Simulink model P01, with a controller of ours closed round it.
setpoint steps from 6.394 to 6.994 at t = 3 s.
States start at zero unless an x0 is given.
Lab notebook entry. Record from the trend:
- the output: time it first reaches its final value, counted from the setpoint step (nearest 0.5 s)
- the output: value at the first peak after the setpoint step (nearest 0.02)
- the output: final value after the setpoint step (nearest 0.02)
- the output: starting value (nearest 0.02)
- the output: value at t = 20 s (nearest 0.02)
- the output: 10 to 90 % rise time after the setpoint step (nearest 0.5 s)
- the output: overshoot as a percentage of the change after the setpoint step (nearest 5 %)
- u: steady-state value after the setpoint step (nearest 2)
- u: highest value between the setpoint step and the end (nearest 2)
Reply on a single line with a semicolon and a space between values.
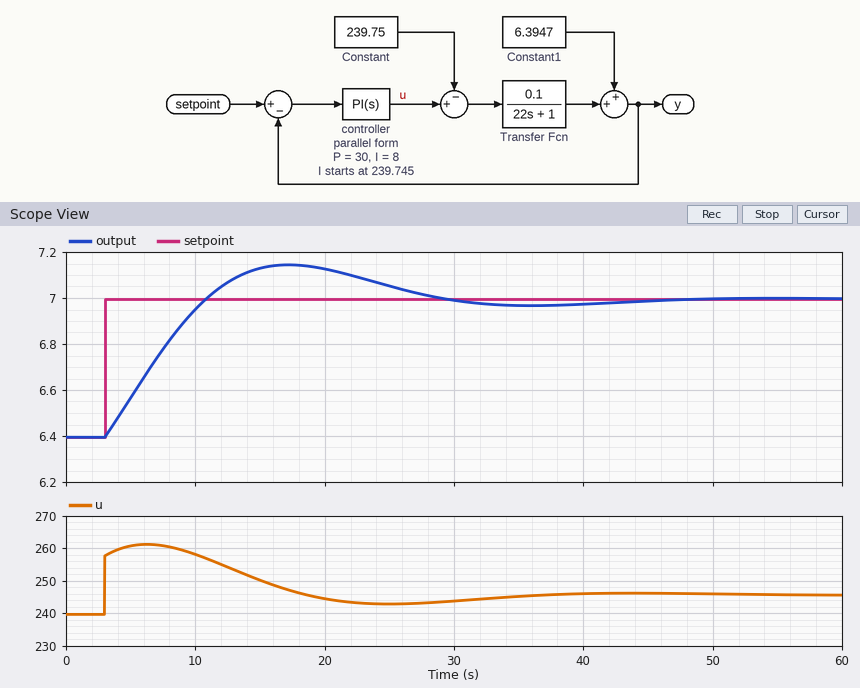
8.0 s; 7.14; 7.00; 6.40; 7.12; 6.0 s; 25 %; 246; 262
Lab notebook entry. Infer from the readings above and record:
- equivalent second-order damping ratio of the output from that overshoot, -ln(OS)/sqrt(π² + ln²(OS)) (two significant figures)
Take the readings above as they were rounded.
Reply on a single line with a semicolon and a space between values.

0.40
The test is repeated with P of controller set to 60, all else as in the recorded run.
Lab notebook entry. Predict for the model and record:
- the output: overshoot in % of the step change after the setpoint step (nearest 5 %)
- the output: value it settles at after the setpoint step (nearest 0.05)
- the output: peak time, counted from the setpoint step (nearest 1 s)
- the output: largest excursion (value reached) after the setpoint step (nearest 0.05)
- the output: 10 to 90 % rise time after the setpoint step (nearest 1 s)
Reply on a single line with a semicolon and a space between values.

10 %; 7.00; 13 s; 7.05; 5 s
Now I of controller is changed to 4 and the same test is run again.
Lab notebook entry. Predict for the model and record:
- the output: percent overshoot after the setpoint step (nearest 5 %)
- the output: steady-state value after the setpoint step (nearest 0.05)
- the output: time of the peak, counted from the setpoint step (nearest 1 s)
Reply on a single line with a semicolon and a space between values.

15 %; 7.00; 20 s
